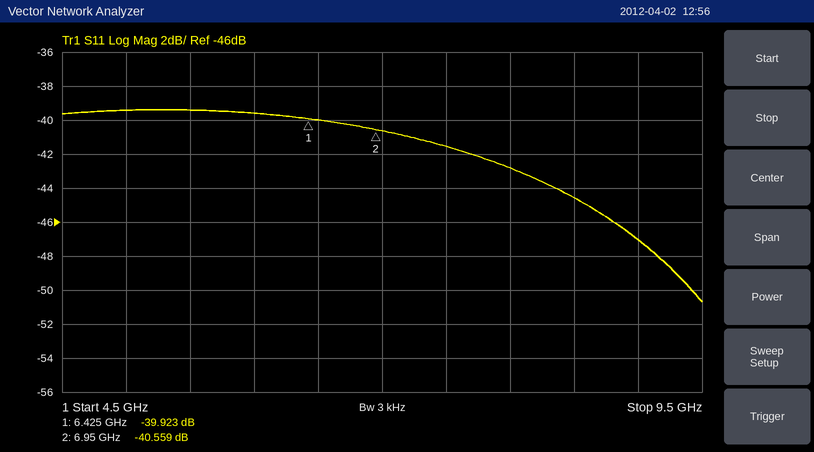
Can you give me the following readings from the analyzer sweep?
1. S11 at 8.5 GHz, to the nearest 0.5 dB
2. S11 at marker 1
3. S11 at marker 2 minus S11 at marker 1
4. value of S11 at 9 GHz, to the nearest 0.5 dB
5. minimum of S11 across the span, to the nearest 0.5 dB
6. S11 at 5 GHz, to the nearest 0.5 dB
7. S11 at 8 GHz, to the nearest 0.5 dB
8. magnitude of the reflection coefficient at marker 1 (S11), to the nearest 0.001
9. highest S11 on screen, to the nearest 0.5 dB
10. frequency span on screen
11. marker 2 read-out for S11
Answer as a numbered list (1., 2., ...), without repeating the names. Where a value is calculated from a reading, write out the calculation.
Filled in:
1. -44.5 dB
2. -39.923 dB
3. -40.559 − (-39.923) = -0.636 dB
4. -47.0 dB
5. -50.5 dB
6. -39.5 dB
7. -43.0 dB
8. 10^(-39.923/20) ≈ 0.010
9. -39.5 dB
10. 5 GHz
11. -40.559 dB
